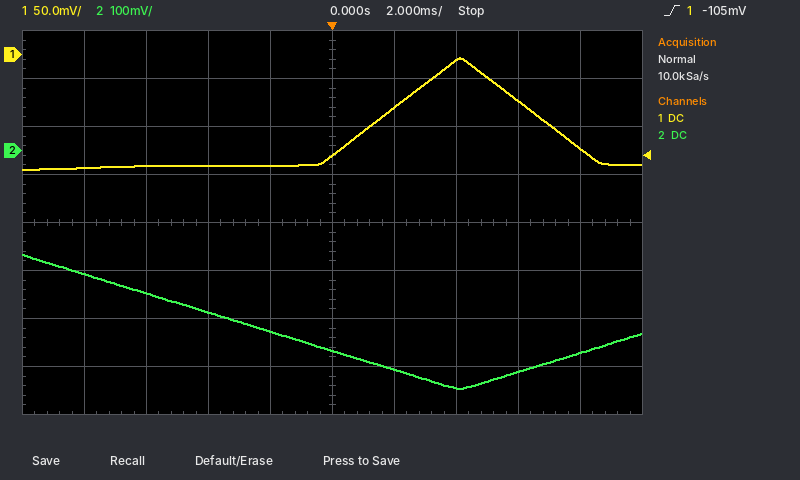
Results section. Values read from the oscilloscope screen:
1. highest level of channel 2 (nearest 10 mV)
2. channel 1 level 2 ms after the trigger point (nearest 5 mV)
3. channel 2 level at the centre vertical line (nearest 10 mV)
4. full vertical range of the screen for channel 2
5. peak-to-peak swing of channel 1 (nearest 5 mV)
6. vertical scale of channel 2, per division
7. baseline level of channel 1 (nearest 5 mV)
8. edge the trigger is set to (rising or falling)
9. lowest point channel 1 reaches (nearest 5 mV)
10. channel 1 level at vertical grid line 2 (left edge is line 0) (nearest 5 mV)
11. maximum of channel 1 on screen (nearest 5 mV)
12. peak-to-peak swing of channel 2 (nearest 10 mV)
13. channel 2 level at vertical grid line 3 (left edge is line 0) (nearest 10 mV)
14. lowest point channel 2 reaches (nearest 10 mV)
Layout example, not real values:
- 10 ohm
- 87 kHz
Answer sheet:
- -220 mV
- -55 mV
- -420 mV
- 800 mV
- 115 mV
- 100 mV
- -115 mV
- rising
- -120 mV
- -115 mV
- -5 mV
- 280 mV
- -340 mV
- -500 mV
